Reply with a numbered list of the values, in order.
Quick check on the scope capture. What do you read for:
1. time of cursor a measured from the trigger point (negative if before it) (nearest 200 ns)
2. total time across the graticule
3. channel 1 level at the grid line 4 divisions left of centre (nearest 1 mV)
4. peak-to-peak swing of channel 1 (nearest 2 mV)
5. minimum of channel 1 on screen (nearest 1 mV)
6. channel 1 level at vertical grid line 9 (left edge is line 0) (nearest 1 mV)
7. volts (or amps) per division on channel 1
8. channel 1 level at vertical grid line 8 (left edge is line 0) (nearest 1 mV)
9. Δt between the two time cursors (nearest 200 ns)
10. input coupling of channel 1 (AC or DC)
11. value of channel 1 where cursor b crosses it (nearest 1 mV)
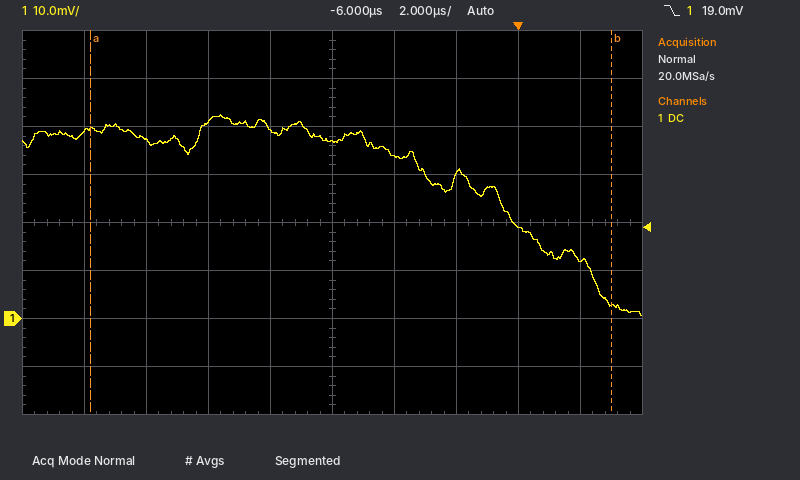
1. -13.8 µs
2. 20 µs
3. 39 mV
4. 42 mV
5. 1 mV
6. 12 mV
7. 10 mV
8. 19 mV
9. 16.8 µs
10. DC
11. 3 mV
